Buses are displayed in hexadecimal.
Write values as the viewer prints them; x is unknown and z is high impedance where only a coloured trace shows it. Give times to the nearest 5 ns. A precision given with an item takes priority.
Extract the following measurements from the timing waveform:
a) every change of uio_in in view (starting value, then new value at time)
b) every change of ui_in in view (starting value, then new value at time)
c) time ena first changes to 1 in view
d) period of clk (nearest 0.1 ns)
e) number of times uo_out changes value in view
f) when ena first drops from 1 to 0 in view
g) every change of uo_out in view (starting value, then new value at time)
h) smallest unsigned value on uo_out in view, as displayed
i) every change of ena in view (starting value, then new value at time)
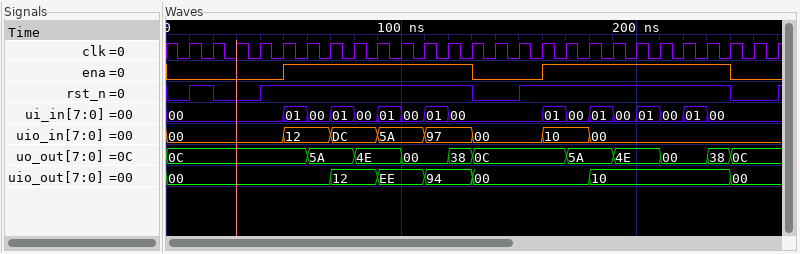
00, 12 at 50 ns, DC at 70 ns, 5A at 90 ns, 97 at 110 ns, 00 at 130 ns, 10 at 160 ns, 00 at 180 ns
00, 01 at 50 ns, 00 at 60 ns, 01 at 70 ns, 00 at 80 ns, 01 at 90 ns, 00 at 100 ns, 01 at 110 ns, 00 at 120 ns, 01 at 160 ns, 00 at 170 ns, 01 at 180 ns, 00 at 190 ns, 01 at 200 ns, 00 at 210 ns, 01 at 220 ns, 00 at 230 ns
50 ns
10 ns
10
130 ns
0C, 5A at 60 ns, 4E at 80 ns, 00 at 100 ns, 38 at 120 ns, 0C at 130 ns, 5A at 170 ns, 4E at 190 ns, 00 at 210 ns, 38 at 230 ns, 0C at 240 ns
00
0, 1 at 50 ns, 0 at 130 ns, 1 at 160 ns, 0 at 240 ns
